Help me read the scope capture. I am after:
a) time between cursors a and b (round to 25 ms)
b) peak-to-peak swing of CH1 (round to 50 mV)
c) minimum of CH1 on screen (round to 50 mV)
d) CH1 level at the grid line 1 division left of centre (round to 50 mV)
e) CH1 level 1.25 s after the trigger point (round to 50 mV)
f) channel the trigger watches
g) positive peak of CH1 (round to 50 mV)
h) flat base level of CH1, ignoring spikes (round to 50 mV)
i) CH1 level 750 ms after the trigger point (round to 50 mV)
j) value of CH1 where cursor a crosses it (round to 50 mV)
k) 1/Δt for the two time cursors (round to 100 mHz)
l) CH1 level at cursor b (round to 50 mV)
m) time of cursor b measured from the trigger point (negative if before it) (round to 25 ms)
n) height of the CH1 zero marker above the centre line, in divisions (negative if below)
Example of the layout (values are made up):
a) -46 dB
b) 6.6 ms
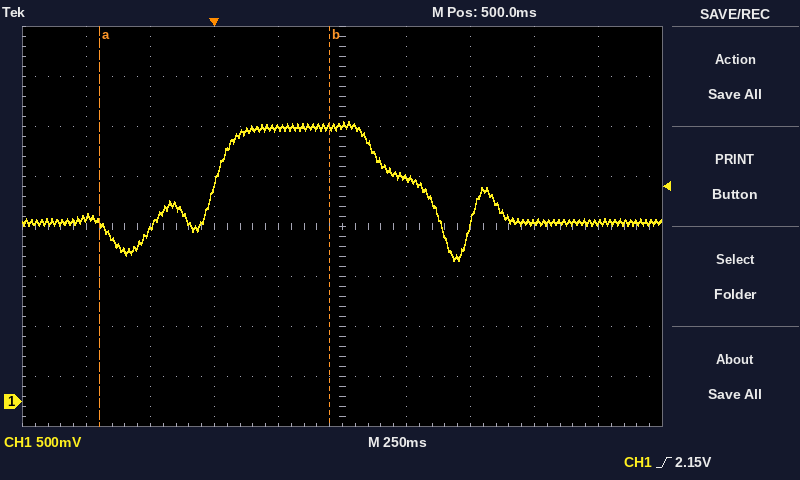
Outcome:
a) 900 ms
b) 1.40 V
c) 1.40 V
d) 2.75 V
e) 1.80 V
f) CH1
g) 2.80 V
h) 1.80 V
i) 2.25 V
j) 1.80 V
k) 1.1 Hz
l) 2.75 V
m) +450 ms
n) -3.5 div
